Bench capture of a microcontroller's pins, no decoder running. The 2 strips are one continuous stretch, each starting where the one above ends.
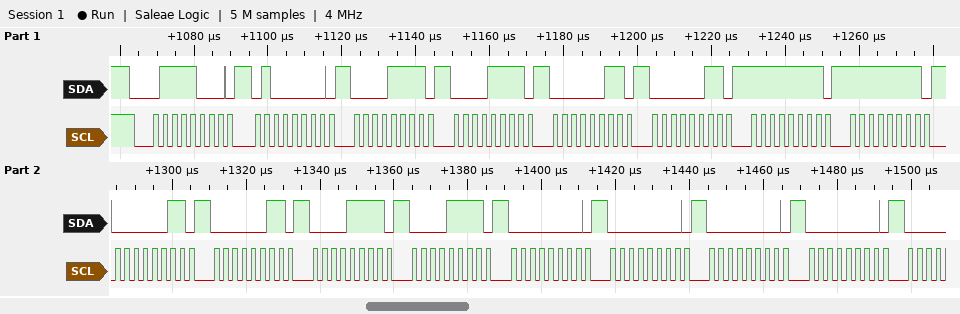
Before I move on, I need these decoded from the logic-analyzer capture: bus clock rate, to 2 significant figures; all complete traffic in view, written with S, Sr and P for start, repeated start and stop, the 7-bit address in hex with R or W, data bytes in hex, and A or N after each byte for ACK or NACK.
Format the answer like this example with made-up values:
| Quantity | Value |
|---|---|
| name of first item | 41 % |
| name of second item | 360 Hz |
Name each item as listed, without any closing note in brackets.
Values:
| Quantity | Value |
|---|---|
| bus clock rate, to 2 significant figures | 400 kHz |
| all complete traffic in view, written with S, Sr and P for start, repeated start and stop, the 7-bit address in hex with R or W, data bytes in hex, and A or N after each byte for ACK or NACK | S 3CW A 40 A 0F A 0F A 03 A 03 A FF A FF A 03 A 03 A 0F A 0F A 00 A 00 A 00 A 00 A |
